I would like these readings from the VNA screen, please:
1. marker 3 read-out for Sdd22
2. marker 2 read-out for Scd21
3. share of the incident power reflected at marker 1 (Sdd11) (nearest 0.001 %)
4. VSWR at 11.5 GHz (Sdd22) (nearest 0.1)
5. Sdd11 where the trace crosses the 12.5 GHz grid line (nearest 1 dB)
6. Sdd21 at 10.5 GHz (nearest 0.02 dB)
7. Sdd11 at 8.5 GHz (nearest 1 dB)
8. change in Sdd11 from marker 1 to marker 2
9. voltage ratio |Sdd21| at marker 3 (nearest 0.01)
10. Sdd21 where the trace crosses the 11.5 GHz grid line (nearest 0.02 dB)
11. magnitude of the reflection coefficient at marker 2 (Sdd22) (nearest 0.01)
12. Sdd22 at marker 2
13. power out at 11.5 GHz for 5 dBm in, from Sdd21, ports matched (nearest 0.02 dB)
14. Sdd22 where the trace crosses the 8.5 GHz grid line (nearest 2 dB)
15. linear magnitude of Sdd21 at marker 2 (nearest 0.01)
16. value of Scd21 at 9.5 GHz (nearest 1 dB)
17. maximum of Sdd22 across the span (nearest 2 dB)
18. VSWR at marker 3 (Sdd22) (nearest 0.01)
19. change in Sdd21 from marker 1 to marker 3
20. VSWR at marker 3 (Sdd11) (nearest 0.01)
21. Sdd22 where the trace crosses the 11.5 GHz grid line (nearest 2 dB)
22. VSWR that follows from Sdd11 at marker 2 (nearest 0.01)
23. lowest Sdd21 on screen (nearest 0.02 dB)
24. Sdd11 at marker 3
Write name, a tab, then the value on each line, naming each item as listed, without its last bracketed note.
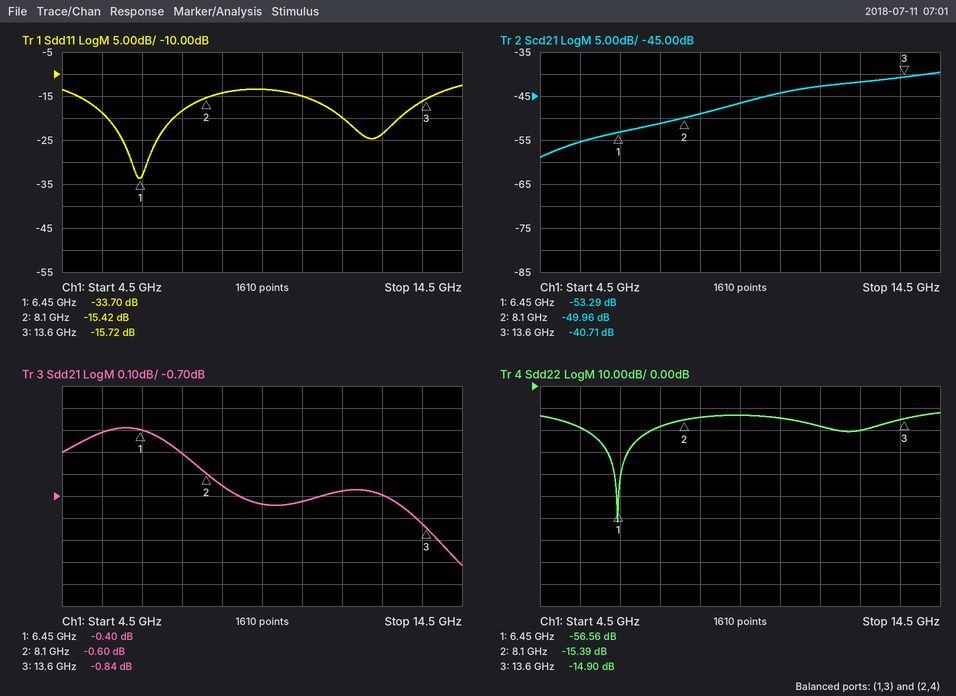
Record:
marker 3 read-out for Sdd22	-14.90 dB
marker 2 read-out for Scd21	-49.96 dB
share of the incident power reflected at marker 1 (Sdd11)	0.043 %
VSWR at 11.5 GHz (Sdd22)	1.3
Sdd11 where the trace crosses the 12.5 GHz grid line	-24 dB
Sdd21 at 10.5 GHz	-0.72 dB
Sdd11 at 8.5 GHz	-14 dB
change in Sdd11 from marker 1 to marker 2	18.28 dB
voltage ratio |Sdd21| at marker 3	0.91
Sdd21 where the trace crosses the 11.5 GHz grid line	-0.68 dB
magnitude of the reflection coefficient at marker 2 (Sdd22)	0.17
Sdd22 at marker 2	-15.39 dB
power out at 11.5 GHz for 5 dBm in, from Sdd21, ports matched	4.32 dBm
Sdd22 where the trace crosses the 8.5 GHz grid line	-14 dB
linear magnitude of Sdd21 at marker 2	0.93
value of Scd21 at 9.5 GHz	-47 dB
maximum of Sdd22 across the span	-12 dB
VSWR at marker 3 (Sdd22)	1.44
change in Sdd21 from marker 1 to marker 3	-0.44 dB
VSWR at marker 3 (Sdd11)	1.39
Sdd22 where the trace crosses the 11.5 GHz grid line	-18 dB
VSWR that follows from Sdd11 at marker 2	1.41
lowest Sdd21 on screen	-1.02 dB
Sdd11 at marker 3	-15.72 dB
